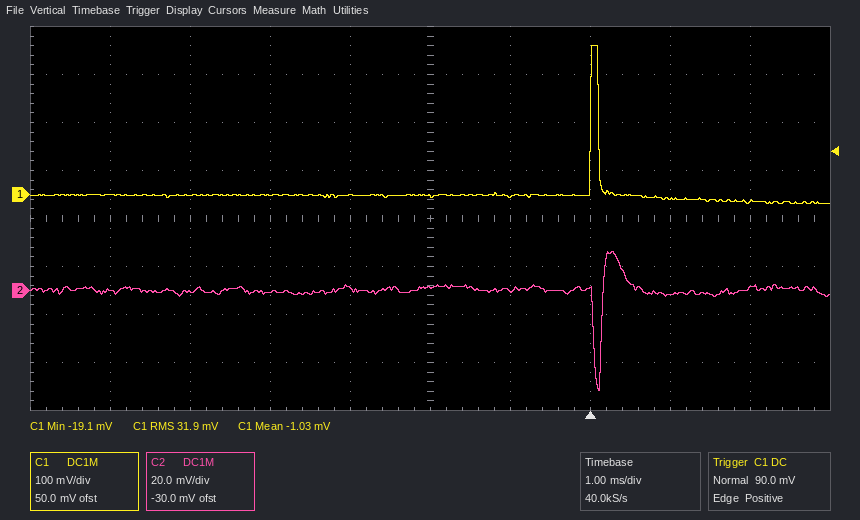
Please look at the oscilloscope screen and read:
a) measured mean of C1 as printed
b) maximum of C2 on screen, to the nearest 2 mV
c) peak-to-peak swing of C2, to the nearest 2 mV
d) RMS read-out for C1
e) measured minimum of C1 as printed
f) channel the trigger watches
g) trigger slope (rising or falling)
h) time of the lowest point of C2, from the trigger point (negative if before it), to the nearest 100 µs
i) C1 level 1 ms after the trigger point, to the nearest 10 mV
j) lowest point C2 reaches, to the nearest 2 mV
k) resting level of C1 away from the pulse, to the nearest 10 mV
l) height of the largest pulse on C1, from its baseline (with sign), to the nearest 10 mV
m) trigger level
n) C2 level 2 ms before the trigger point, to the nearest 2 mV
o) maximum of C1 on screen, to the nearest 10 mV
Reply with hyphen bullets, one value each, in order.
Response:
- -1.03 mV
- 16 mV
- 58 mV
- 31.9 mV
- -19.1 mV
- C1
- rising
- +100 µs
- -10 mV
- -42 mV
- 0 mV
- +310 mV
- 90.0 mV
- 2 mV
- 310 mV
